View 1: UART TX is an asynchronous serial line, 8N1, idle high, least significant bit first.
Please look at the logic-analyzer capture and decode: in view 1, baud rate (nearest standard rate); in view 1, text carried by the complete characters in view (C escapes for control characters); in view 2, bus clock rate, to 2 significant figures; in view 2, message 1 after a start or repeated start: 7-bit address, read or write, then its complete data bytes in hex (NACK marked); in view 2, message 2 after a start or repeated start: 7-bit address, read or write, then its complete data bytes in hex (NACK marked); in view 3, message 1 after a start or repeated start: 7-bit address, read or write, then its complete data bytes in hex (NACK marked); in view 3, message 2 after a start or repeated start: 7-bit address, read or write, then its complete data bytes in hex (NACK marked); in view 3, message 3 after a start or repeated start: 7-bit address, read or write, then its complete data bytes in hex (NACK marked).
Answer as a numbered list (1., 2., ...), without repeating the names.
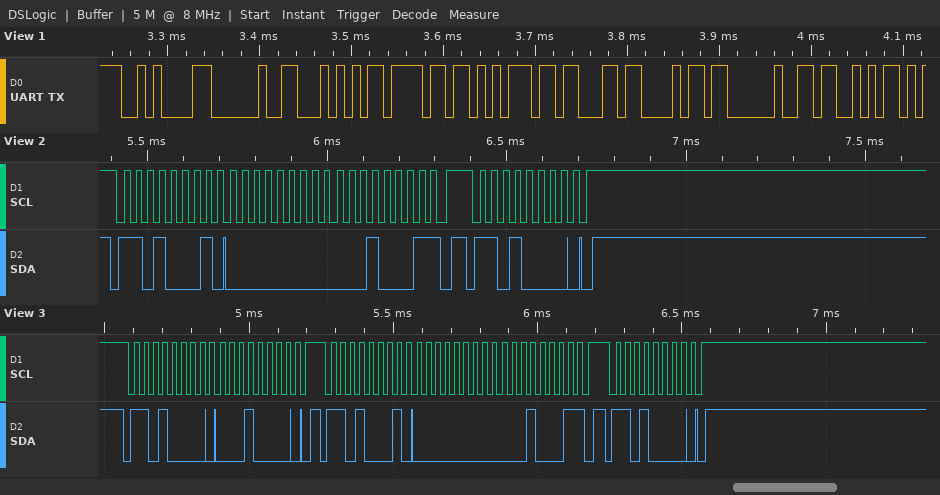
1. 115200 baud
2. "\n Touch S"
3. 31 kHz
4. 0x68 read: 00 11 NACK
5. 0x68 write
6. 0x68 write: 10
7. 0x68 read: 00 11 NACK
8. 0x68 write
